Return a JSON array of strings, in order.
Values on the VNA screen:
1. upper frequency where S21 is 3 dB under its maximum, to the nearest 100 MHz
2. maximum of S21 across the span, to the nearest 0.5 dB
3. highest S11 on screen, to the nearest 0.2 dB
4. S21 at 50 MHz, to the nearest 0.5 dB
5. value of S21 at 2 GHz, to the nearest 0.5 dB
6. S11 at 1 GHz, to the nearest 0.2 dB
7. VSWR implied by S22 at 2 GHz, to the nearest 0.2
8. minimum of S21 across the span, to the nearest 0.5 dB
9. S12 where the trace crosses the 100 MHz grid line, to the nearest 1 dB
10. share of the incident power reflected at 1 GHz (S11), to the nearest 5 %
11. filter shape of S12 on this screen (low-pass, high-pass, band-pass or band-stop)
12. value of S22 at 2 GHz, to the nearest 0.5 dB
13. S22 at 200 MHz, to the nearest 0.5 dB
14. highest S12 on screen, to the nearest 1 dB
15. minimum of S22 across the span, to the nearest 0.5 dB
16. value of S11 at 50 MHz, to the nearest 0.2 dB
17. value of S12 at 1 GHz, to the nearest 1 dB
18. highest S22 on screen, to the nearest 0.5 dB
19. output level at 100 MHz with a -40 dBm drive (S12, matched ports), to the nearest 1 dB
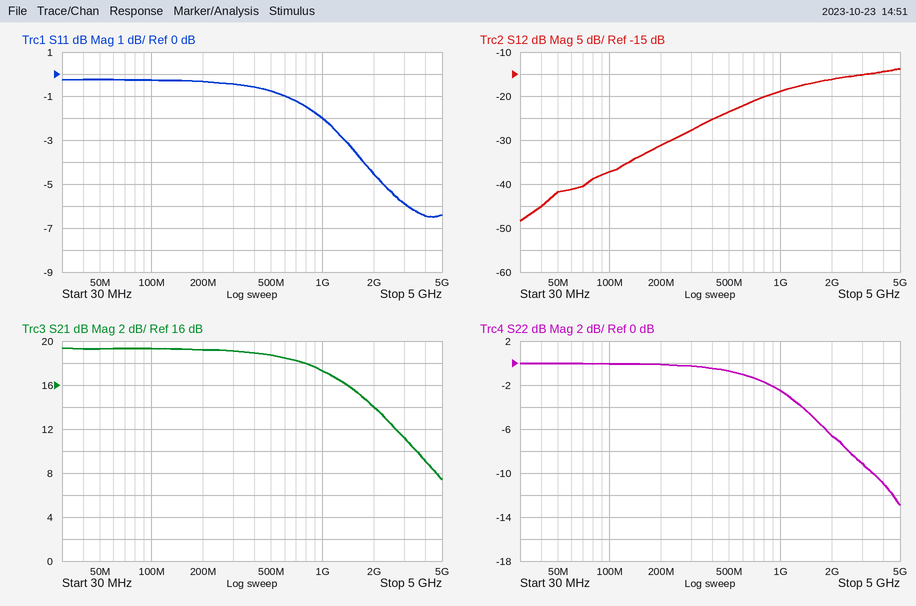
["1.3 GHz", "19.5 dB", "-0.2 dB", "19.5 dB", "14.0 dB", "-2.0 dB", "2.8", "7.5 dB", "-37 dB", "65 %", "high-pass", "-6.5 dB", "0.0 dB", "-14 dB", "-13.0 dB", "-0.2 dB", "-19 dB", "0.0 dB", "-77 dBm"]
